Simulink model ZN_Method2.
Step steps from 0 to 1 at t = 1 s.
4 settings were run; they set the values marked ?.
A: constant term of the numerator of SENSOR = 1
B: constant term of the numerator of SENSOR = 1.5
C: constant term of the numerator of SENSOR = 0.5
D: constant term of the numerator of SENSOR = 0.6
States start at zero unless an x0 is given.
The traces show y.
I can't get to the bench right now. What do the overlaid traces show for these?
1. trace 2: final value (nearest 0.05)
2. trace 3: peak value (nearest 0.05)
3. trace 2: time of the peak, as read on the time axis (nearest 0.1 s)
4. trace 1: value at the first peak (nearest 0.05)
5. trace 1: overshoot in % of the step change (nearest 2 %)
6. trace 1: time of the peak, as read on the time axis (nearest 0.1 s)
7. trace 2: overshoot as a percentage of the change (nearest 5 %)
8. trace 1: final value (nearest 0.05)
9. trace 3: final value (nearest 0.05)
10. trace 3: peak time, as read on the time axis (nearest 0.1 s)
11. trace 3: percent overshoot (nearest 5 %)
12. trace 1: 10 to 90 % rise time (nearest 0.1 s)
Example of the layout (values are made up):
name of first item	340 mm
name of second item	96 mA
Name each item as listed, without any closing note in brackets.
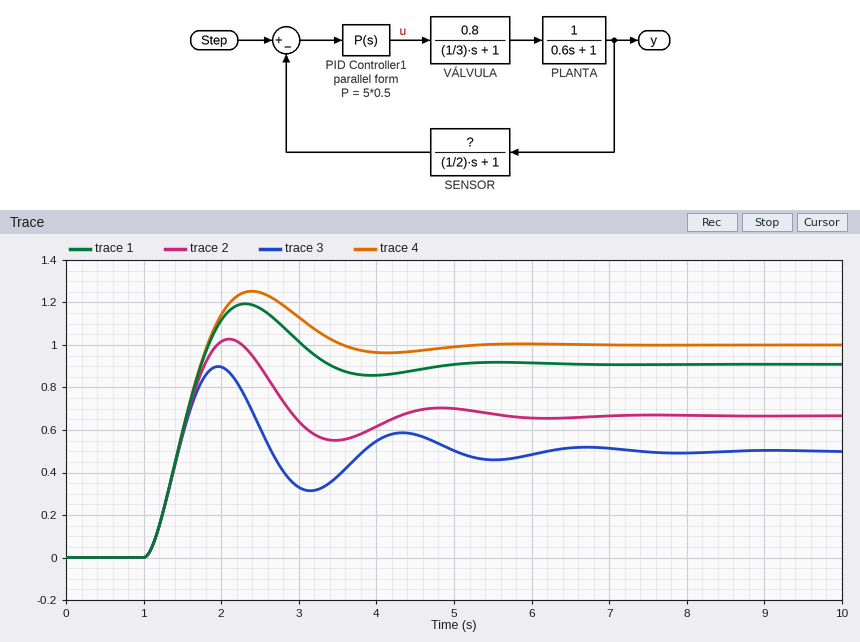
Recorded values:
trace 2: final value	0.65
trace 3: peak value	0.90
trace 2: time of the peak, as read on the time axis	2.1 s
trace 1: value at the first peak	1.20
trace 1: overshoot in % of the step change	32 %
trace 1: time of the peak, as read on the time axis	2.3 s
trace 2: overshoot as a percentage of the change	55 %
trace 1: final value	0.90
trace 3: final value	0.50
trace 3: peak time, as read on the time axis	2.0 s
trace 3: percent overshoot	80 %
trace 1: 10 to 90 % rise time	0.5 s
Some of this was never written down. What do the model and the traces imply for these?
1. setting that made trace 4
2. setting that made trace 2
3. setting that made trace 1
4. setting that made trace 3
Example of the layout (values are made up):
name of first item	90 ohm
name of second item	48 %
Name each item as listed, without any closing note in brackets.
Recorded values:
setting that made trace 4	C
setting that made trace 2	A
setting that made trace 1	D
setting that made trace 3	B
